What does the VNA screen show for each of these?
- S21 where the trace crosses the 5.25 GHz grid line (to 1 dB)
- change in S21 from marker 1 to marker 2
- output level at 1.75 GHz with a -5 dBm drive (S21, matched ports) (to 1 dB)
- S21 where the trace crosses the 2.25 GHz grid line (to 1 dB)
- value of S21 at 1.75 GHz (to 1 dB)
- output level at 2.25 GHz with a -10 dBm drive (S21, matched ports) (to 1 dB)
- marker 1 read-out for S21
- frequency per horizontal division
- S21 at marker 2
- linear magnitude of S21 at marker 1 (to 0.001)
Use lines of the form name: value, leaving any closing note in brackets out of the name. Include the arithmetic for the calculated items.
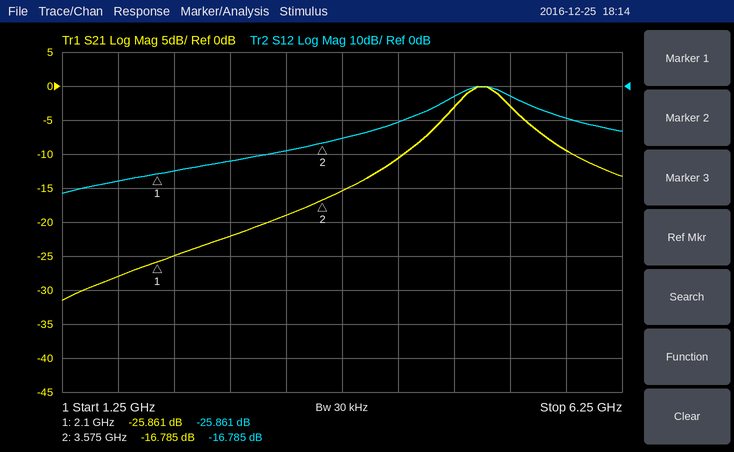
S21 where the trace crosses the 5.25 GHz grid line: -3 dB
change in S21 from marker 1 to marker 2: -16.785 − (-25.861) = 9.076 dB
output level at 1.75 GHz with a -5 dBm drive (S21, matched ports): -5 dBm + (-28 dB) = -33 dBm
S21 where the trace crosses the 2.25 GHz grid line: -25 dB
value of S21 at 1.75 GHz: -28 dB
output level at 2.25 GHz with a -10 dBm drive (S21, matched ports): -10 dBm + (-25 dB) = -35 dBm
marker 1 read-out for S21: -25.861 dB
frequency per horizontal division: 500 MHz
S21 at marker 2: -16.785 dB
linear magnitude of S21 at marker 1: 10^(-25.861/20) ≈ 0.051
